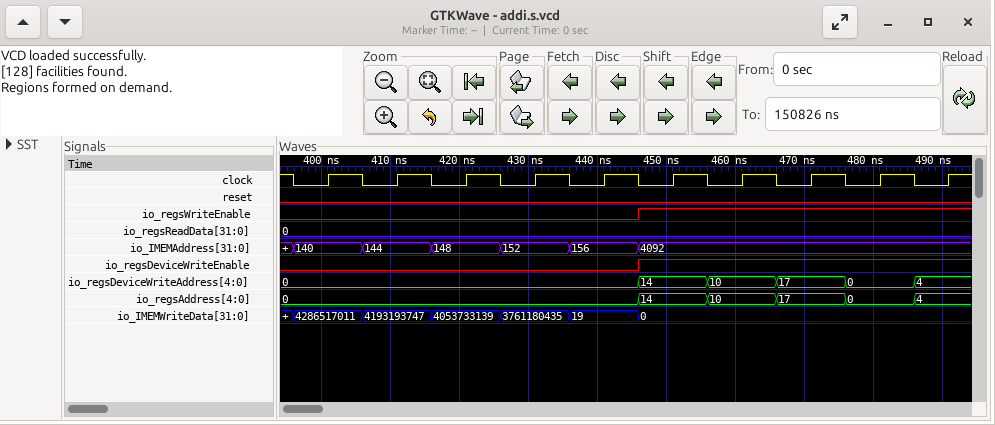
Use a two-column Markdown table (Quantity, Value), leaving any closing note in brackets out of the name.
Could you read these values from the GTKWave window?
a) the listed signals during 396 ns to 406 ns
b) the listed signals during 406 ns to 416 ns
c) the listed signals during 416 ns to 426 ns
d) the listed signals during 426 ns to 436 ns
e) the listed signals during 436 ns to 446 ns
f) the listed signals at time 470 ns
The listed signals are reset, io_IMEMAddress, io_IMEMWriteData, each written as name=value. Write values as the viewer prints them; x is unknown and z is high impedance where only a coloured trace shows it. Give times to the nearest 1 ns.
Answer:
| Quantity | Value |
|---|---|
| the listed signals during 396 ns to 406 ns | reset=0, io_IMEMAddress=140, io_IMEMWriteData=4286517011 |
| the listed signals during 406 ns to 416 ns | reset=0, io_IMEMAddress=144, io_IMEMWriteData=4193193747 |
| the listed signals during 416 ns to 426 ns | reset=0, io_IMEMAddress=148, io_IMEMWriteData=4053733139 |
| the listed signals during 426 ns to 436 ns | reset=0, io_IMEMAddress=152, io_IMEMWriteData=3761180435 |
| the listed signals during 436 ns to 446 ns | reset=0, io_IMEMAddress=156, io_IMEMWriteData=19 |
| the listed signals at time 470 ns | reset=0, io_IMEMAddress=4092, io_IMEMWriteData=0 |
